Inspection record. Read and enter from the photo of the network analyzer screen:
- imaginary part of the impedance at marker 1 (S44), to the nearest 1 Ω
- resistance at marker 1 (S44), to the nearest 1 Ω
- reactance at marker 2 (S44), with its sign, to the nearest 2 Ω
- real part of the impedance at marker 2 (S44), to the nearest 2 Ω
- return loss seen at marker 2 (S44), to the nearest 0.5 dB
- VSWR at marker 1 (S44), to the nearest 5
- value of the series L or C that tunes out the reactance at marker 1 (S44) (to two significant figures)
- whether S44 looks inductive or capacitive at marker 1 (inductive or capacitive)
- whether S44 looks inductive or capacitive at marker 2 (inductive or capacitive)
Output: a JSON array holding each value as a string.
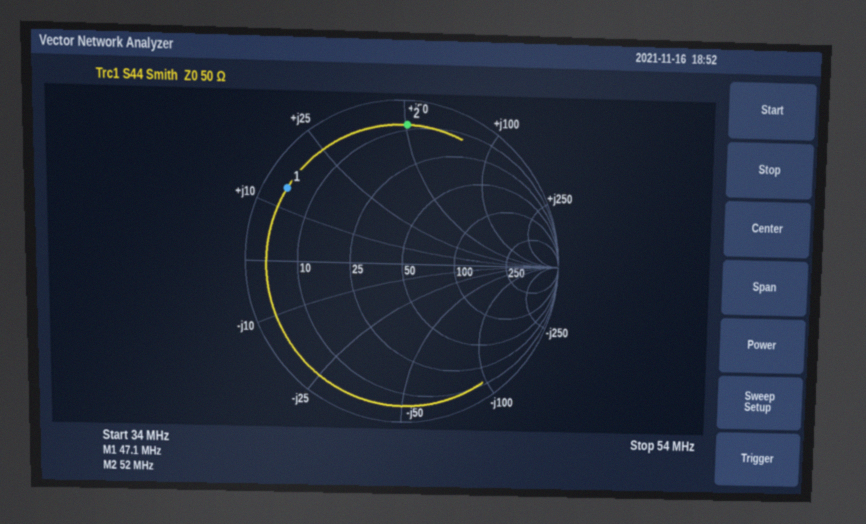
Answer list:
["+14 Ω", "4 Ω", "+50 Ω", "8 Ω", "1.5 dB", "15", "240 pF", "inductive", "inductive"]
